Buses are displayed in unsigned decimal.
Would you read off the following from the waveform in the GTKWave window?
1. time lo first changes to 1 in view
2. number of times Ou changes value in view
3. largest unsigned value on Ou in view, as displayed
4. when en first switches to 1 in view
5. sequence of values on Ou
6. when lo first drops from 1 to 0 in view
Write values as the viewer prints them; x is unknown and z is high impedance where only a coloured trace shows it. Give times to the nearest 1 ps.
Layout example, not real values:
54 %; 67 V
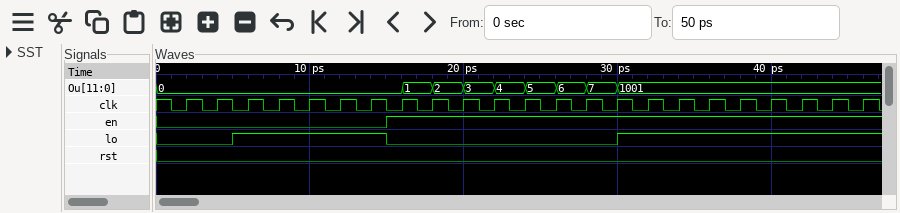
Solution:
5 ps; 8; 1001; 15 ps; 0, 1, 2, 3, 4, 5, 6, 7, 1001; 15 ps
